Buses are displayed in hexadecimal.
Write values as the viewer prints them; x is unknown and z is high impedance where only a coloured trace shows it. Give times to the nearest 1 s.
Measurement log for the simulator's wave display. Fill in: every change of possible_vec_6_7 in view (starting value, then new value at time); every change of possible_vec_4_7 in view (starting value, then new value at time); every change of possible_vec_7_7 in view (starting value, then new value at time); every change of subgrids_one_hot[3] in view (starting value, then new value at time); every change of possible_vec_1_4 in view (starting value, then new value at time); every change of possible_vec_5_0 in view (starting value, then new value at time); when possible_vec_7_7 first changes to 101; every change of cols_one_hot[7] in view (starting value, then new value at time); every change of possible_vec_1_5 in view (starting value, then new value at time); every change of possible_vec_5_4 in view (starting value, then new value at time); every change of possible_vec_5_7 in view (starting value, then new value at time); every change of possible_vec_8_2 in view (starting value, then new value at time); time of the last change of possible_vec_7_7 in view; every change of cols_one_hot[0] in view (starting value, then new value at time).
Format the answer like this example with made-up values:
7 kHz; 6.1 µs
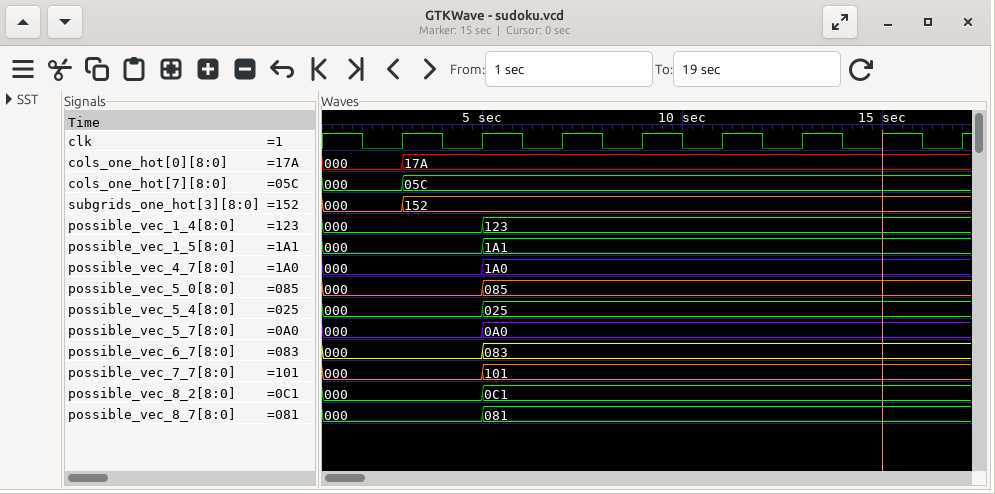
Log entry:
000, 083 at 5 s; 000, 1A0 at 5 s; 000, 101 at 5 s; 000, 152 at 3 s; 000, 123 at 5 s; 000, 085 at 5 s; 5 s; 000, 05C at 3 s; 000, 1A1 at 5 s; 000, 025 at 5 s; 000, 0A0 at 5 s; 000, 0C1 at 5 s; 5 s; 000, 17A at 3 s
